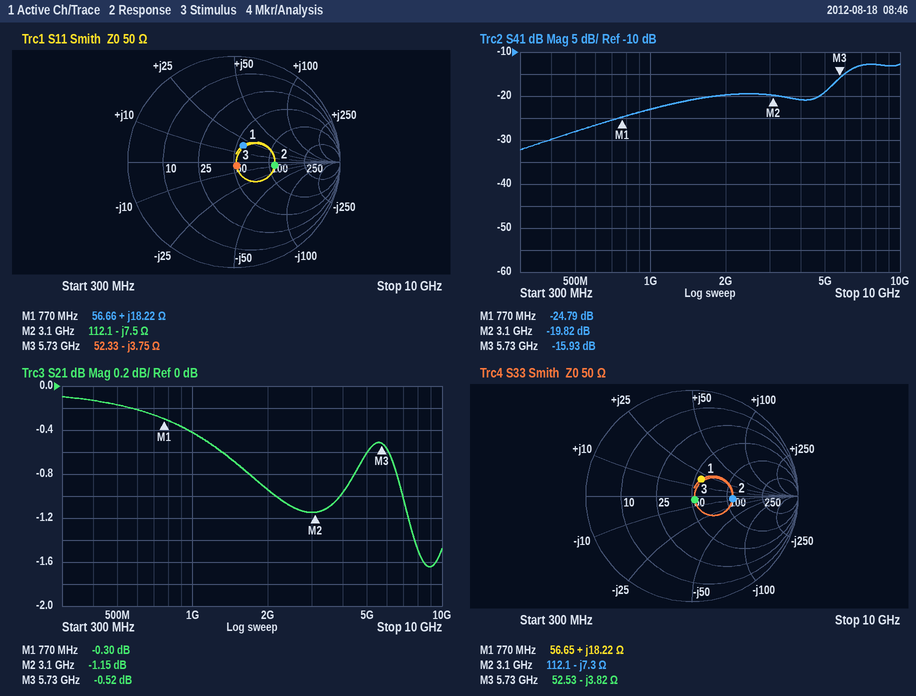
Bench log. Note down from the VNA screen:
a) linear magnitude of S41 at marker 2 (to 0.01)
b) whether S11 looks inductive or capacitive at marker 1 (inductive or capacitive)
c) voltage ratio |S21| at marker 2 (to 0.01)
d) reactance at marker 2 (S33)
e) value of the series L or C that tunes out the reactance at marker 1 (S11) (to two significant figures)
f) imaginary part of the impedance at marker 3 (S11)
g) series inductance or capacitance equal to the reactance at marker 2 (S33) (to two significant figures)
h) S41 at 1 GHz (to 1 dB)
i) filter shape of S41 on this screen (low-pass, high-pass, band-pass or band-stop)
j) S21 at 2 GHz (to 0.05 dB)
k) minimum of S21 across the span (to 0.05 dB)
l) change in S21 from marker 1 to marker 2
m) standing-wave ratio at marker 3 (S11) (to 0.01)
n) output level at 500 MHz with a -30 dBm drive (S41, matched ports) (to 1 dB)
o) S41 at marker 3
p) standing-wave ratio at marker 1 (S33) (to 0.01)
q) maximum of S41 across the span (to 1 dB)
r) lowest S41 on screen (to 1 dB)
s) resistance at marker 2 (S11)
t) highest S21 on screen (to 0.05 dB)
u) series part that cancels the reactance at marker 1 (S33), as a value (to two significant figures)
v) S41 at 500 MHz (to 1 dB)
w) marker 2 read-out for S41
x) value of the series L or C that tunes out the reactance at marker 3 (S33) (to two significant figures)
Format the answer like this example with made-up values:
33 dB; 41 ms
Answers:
0.10; inductive; 0.88; -7.3 Ω; 11 pF; -3.75 Ω; 7.0 pF; -23 dB; high-pass; -0.95 dB; -1.65 dB; -0.85 dB; 1.09; -58 dBm; -15.93 dB; 1.44; -13 dB; -32 dB; 112.1 Ω; -0.10 dB; 11 pF; -28 dB; -19.82 dB; 110 pH
